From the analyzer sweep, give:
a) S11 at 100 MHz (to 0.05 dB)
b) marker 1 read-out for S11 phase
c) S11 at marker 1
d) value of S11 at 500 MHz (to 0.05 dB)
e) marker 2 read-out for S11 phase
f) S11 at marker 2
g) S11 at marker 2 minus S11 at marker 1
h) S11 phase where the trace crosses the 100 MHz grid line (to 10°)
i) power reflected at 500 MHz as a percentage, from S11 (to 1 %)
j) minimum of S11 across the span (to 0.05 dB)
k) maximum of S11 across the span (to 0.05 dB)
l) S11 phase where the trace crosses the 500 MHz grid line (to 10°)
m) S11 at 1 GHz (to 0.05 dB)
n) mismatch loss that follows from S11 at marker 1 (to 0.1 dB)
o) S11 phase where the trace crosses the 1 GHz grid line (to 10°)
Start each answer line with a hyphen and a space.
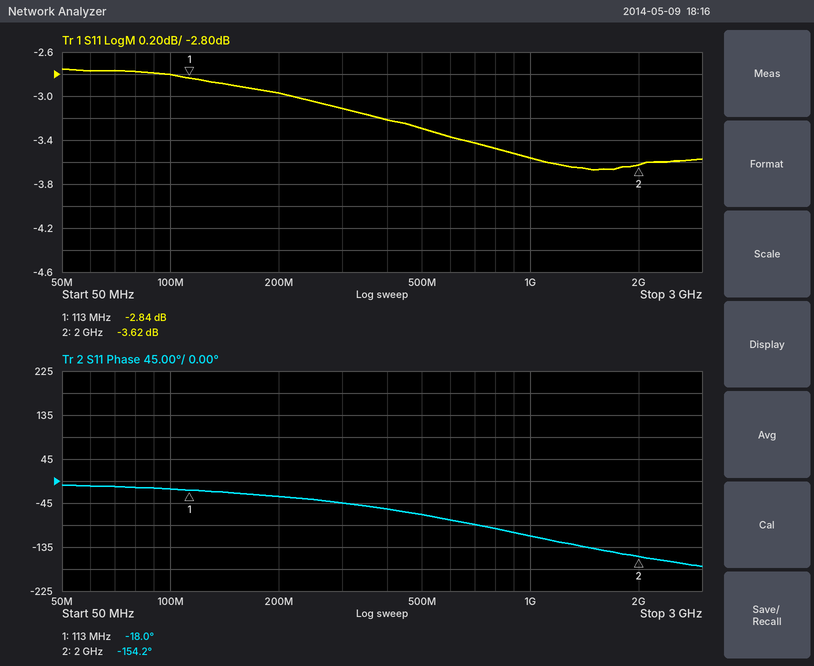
- -2.80 dB
- -18.0°
- -2.84 dB
- -3.30 dB
- -154.2°
- -3.62 dB
- -0.78 dB
- -20°
- 47 %
- -3.65 dB
- -2.75 dB
- -70°
- -3.55 dB
- 3.2 dB
- -110°
